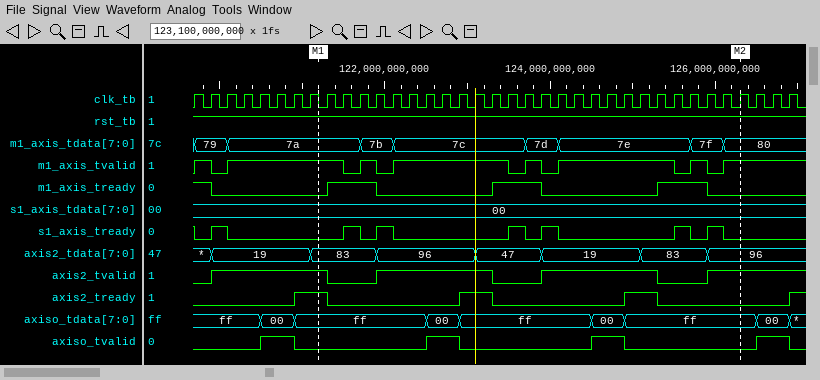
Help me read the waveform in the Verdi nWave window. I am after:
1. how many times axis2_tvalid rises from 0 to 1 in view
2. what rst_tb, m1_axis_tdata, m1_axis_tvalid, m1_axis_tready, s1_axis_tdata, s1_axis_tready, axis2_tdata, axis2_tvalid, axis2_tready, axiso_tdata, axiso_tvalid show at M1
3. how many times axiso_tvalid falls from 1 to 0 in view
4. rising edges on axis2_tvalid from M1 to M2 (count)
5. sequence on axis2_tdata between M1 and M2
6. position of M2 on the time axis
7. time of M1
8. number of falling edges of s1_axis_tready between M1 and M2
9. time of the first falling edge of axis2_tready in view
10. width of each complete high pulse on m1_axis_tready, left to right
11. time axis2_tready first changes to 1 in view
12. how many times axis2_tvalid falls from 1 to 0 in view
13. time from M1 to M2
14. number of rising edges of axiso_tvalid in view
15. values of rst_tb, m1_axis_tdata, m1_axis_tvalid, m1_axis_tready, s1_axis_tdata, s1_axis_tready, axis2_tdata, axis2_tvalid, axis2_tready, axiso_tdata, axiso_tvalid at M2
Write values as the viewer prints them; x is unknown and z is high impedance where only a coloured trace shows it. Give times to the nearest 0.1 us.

4
rst_tb=1, m1_axis_tdata=7a, m1_axis_tvalid=1, m1_axis_tready=0, s1_axis_tdata=00, s1_axis_tready=0, axis2_tdata=83, axis2_tvalid=1, axis2_tready=1, axiso_tdata=ff, axiso_tvalid=0
4
3
83, 96, 47, 19, 83, 96
126.3 us
121.2 us
6
121.3 us
0.6 us, 0.6 us, 0.6 us
120.9 us
3
5.1 us
4
rst_tb=1, m1_axis_tdata=80, m1_axis_tvalid=1, m1_axis_tready=0, s1_axis_tdata=00, s1_axis_tready=0, axis2_tdata=96, axis2_tvalid=1, axis2_tready=0, axiso_tdata=ff, axiso_tvalid=0
